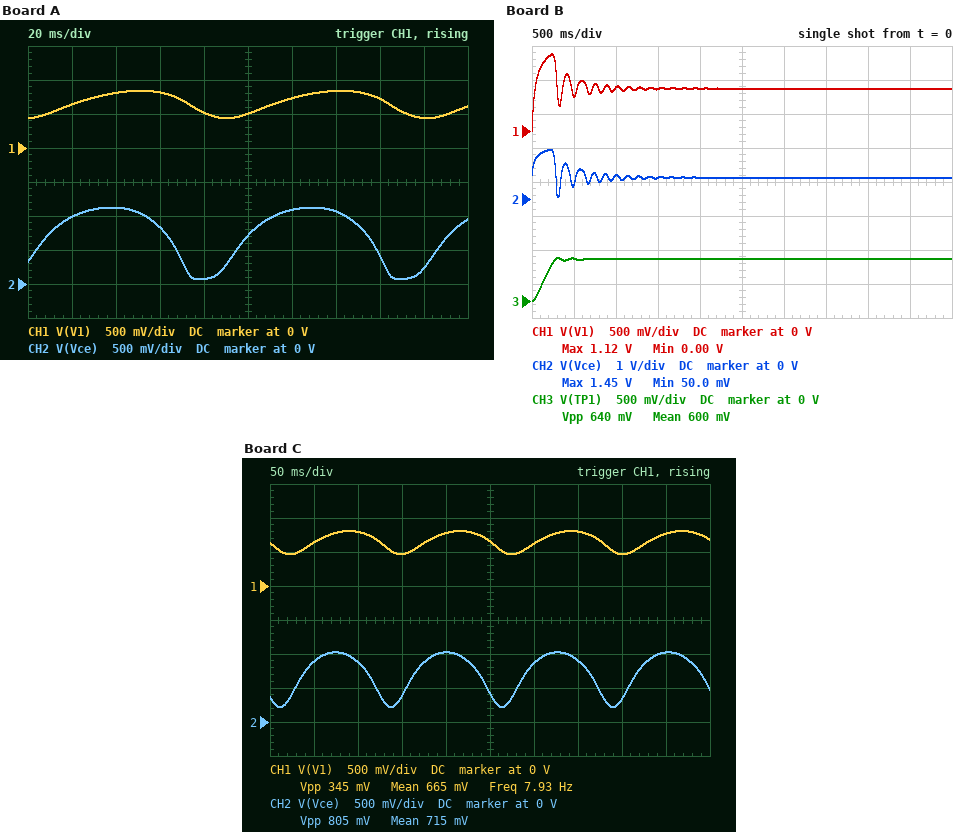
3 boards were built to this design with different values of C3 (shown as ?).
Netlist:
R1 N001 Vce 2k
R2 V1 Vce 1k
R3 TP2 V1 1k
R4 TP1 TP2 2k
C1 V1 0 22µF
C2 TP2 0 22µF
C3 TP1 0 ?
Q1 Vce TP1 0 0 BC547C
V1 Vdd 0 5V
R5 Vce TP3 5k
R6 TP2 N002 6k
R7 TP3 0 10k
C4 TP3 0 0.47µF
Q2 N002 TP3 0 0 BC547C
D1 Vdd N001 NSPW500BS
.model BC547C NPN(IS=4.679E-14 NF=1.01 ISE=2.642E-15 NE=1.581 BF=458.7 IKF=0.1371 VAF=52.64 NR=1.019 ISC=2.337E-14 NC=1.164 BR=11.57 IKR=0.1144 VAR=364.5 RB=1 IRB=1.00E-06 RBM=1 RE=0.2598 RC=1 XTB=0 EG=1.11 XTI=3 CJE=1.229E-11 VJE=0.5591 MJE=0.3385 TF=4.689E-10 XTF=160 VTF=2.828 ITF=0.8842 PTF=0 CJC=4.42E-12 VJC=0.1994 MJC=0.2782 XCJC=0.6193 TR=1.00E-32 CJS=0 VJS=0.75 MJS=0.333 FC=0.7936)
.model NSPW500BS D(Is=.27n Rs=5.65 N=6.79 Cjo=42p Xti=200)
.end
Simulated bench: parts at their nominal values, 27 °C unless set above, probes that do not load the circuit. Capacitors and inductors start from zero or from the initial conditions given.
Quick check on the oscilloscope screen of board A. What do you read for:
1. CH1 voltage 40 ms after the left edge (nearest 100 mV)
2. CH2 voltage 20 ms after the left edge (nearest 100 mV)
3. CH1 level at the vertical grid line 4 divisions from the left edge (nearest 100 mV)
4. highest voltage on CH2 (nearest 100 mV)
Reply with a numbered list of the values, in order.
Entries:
1. 800 mV
2. 1.0 V
3. 500 mV
4. 1.1 V
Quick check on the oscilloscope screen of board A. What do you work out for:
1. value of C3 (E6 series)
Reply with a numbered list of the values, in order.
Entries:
1. 15 µF
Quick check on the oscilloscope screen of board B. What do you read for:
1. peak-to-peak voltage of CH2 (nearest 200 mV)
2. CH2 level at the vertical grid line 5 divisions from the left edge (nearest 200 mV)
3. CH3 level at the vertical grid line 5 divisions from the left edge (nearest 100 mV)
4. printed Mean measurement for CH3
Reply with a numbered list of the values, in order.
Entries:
1. 1.4 V
2. 600 mV
3. 600 mV
4. 600 mV
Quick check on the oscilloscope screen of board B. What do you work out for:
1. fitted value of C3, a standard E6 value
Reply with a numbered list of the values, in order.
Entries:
1. 68 µF
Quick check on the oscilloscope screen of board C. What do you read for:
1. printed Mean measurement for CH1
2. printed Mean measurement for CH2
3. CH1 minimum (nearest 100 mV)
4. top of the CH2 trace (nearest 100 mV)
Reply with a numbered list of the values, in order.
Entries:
1. 665 mV
2. 715 mV
3. 500 mV
4. 1.0 V
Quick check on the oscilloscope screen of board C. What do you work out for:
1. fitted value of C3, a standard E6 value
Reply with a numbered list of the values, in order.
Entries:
1. 33 µF
